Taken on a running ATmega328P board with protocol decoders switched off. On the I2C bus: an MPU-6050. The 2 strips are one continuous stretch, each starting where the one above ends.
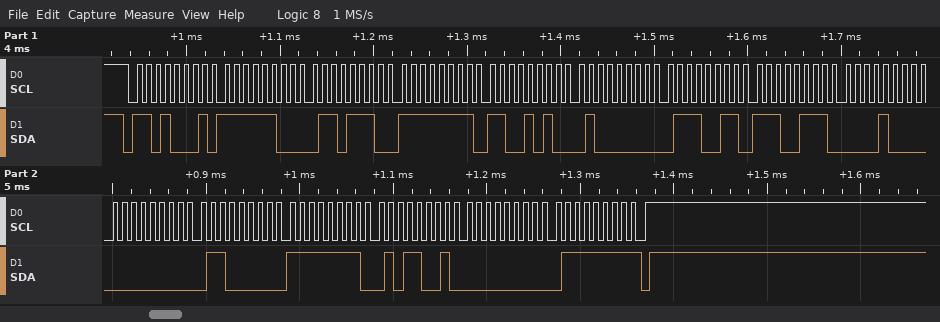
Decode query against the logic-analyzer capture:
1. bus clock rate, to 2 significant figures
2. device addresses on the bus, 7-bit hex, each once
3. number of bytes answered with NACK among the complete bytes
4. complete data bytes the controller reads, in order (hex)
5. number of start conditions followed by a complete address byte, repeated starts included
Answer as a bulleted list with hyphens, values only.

- 100 kHz
- 0x68
- 1
- FC 6E FF CA 40 73 E7 08 00 60 FF 59 00 7F
- 1
